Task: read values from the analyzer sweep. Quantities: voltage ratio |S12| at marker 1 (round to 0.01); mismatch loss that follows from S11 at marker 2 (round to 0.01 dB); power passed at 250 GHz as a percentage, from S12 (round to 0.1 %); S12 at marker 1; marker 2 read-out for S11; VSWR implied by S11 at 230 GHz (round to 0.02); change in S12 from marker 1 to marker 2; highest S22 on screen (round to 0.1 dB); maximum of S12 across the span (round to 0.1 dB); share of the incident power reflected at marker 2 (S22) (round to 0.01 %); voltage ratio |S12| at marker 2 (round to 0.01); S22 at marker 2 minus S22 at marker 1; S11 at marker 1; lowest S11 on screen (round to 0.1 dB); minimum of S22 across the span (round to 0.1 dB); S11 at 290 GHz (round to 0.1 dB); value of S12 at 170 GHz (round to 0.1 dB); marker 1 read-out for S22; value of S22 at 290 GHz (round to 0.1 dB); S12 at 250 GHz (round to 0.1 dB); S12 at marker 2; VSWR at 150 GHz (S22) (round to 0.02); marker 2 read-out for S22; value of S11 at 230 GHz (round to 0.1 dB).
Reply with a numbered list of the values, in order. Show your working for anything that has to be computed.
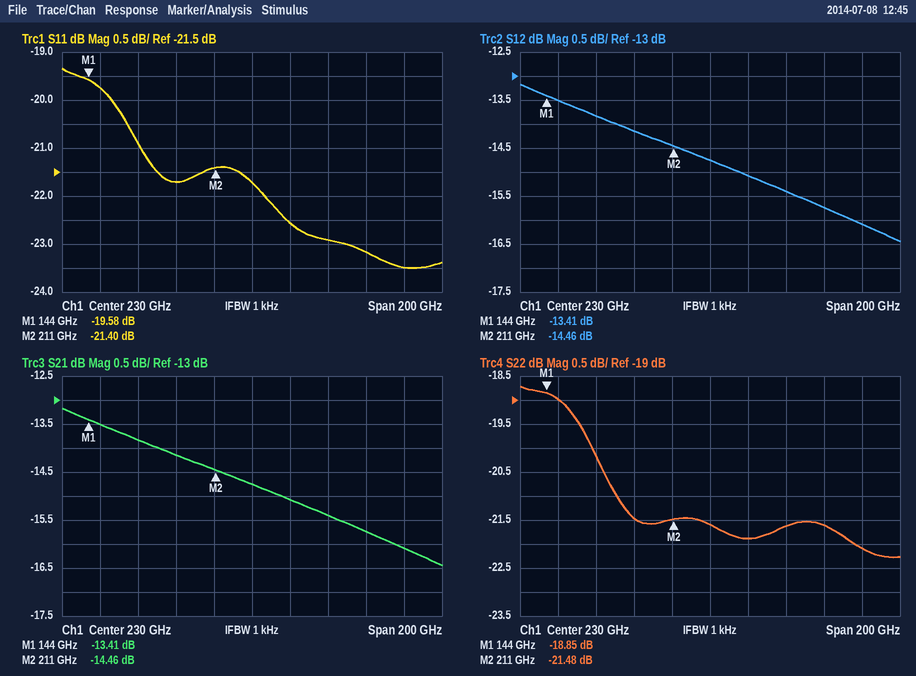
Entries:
1. 10^(-13.41/20) ≈ 0.21
2. −10 log10(1 − 10^(-21.4/10)) ≈ 0.03 dB
3. 10^(-15.1/10) ≈ 3.1 %
4. -13.41 dB
5. -21.40 dB
6. |Γ| = 10^(-21.7/20) = 0.0822; VSWR = (1 + 0.0822)/(1 − 0.0822) ≈ 1.18
7. -14.46 − (-13.41) = -1.05 dB
8. -18.7 dB
9. -13.2 dB
10. 10^(-21.48/10) ≈ 0.71 %
11. 10^(-14.46/20) ≈ 0.19
12. -21.48 − (-18.85) = -2.63 dB
13. -19.58 dB
14. -23.5 dB
15. -22.3 dB
16. -23.2 dB
17. -13.8 dB
18. -18.85 dB
19. -21.6 dB
20. -15.1 dB
21. -14.46 dB
22. |Γ| = 10^(-19/20) = 0.1122; VSWR = (1 + 0.1122)/(1 − 0.1122) ≈ 1.25, so 1.26 to the nearest 0.02
23. -21.48 dB
24. -21.7 dB
